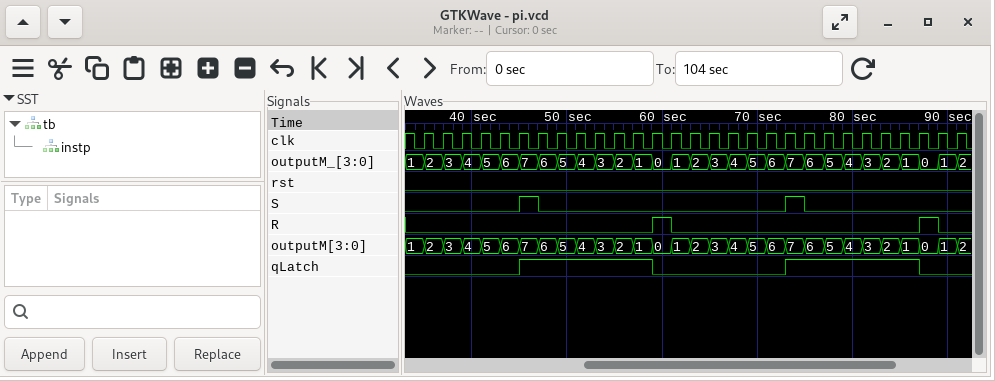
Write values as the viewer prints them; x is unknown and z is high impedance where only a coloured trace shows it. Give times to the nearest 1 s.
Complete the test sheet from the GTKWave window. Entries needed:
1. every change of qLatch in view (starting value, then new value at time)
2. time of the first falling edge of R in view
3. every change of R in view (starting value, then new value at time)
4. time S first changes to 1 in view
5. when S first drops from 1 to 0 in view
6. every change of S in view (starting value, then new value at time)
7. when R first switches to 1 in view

0, 1 at 45 s, 0 at 59 s, 1 at 73 s, 0 at 87 s
61 s
0, 1 at 59 s, 0 at 61 s, 1 at 87 s, 0 at 89 s
45 s
47 s
0, 1 at 45 s, 0 at 47 s, 1 at 73 s, 0 at 75 s
59 s
